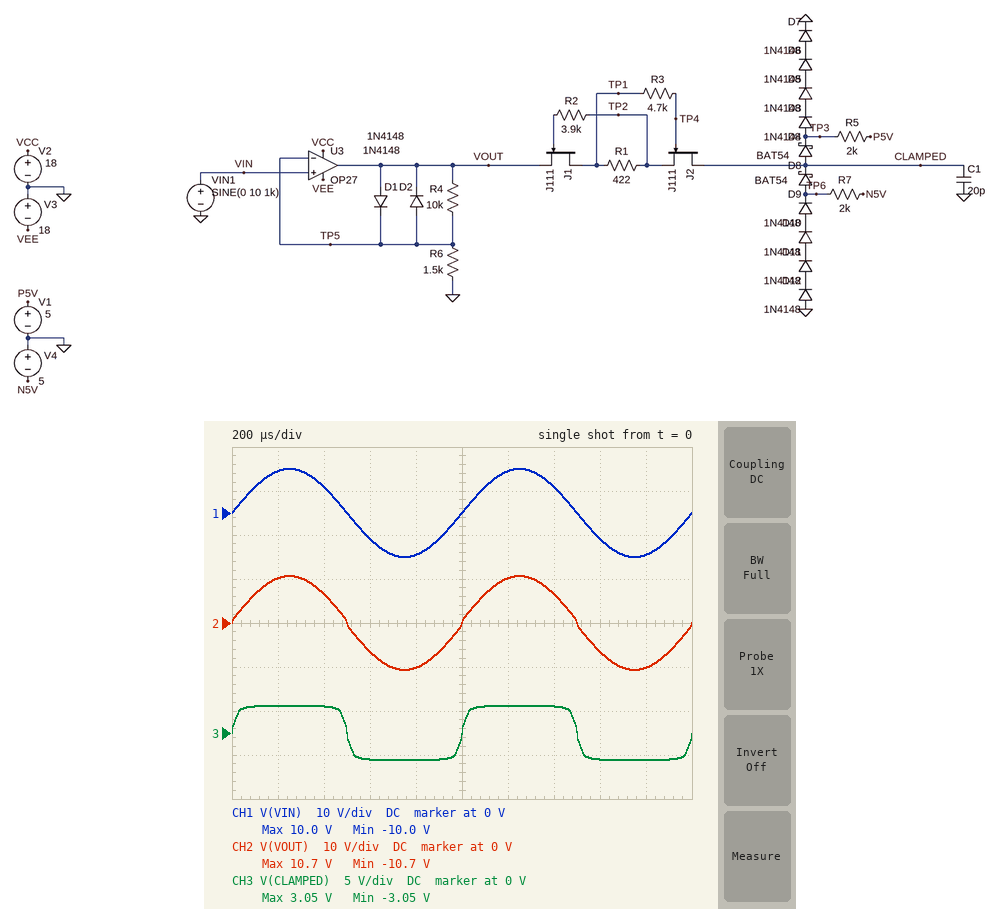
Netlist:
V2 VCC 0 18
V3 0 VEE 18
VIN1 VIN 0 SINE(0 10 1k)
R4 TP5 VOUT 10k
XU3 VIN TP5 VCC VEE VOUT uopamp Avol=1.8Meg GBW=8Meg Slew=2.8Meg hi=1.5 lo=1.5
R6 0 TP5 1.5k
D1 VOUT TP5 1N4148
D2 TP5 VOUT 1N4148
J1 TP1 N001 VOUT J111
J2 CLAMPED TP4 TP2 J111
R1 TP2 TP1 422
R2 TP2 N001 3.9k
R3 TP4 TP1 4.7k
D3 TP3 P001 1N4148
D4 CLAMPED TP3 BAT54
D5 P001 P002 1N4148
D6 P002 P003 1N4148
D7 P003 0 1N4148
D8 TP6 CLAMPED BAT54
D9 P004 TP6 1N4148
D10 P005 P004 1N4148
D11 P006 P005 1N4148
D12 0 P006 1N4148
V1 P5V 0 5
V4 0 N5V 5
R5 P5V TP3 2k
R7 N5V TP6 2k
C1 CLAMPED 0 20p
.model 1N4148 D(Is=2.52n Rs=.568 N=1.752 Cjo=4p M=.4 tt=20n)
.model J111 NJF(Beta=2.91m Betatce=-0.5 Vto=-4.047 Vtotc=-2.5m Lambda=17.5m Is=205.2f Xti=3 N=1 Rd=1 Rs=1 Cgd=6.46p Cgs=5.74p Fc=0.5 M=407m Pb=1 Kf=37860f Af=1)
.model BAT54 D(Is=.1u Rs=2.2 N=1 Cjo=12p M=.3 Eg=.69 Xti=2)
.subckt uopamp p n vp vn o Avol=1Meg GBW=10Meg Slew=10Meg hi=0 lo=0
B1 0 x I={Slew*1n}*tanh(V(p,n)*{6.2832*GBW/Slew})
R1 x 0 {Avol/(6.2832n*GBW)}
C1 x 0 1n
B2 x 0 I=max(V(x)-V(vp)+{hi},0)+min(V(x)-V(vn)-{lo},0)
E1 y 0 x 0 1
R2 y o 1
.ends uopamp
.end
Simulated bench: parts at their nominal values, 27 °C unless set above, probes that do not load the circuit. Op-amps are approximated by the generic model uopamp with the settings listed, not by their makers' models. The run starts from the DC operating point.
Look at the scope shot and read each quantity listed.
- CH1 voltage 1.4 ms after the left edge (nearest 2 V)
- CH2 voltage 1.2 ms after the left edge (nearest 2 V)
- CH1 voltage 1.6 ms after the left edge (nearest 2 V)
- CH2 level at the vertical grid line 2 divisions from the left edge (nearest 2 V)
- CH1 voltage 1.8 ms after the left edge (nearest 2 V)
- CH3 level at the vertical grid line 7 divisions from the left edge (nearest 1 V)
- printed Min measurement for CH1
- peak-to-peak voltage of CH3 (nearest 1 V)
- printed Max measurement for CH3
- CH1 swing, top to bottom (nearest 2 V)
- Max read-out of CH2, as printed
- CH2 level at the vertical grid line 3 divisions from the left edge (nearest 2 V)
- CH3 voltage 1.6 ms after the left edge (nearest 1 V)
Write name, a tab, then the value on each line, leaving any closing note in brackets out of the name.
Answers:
CH1 voltage 1.4 ms after the left edge	6 V
CH2 voltage 1.2 ms after the left edge	10 V
CH1 voltage 1.6 ms after the left edge	-6 V
CH2 level at the vertical grid line 2 divisions from the left edge	6 V
CH1 voltage 1.8 ms after the left edge	-10 V
CH3 level at the vertical grid line 7 divisions from the left edge	3 V
printed Min measurement for CH1	-10.0 V
peak-to-peak voltage of CH3	6 V
printed Max measurement for CH3	3.05 V
CH1 swing, top to bottom	20 V
Max read-out of CH2, as printed	10.7 V
CH2 level at the vertical grid line 3 divisions from the left edge	-6 V
CH3 voltage 1.6 ms after the left edge	-3 V
